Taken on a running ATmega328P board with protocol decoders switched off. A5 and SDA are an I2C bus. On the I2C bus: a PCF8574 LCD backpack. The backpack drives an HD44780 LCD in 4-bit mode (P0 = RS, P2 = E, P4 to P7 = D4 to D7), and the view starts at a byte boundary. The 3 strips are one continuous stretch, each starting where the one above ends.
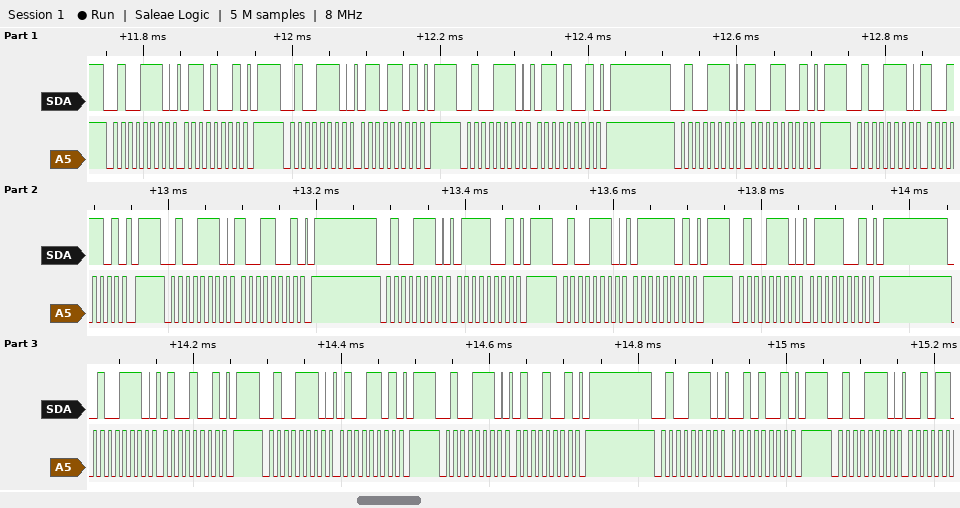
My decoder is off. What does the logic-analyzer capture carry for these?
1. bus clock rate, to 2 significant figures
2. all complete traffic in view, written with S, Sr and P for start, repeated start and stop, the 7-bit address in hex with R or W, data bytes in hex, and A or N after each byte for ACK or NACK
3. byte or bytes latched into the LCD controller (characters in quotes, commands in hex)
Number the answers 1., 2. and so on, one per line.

1. 100 kHz
2. S 27W A 69 A P S 27W A 6D A P S 27W A 69 A P S 27W A 99 A P S 27W A 9D A P S 27W A 99 A P S 27W A 79 A P S 27W A 7D A P S 27W A 79 A P S 27W A 49 A P S 27W A 4D A P S 27W A 49 A P S 27W A 29 A P S 27W A
3. 'i' 't'
